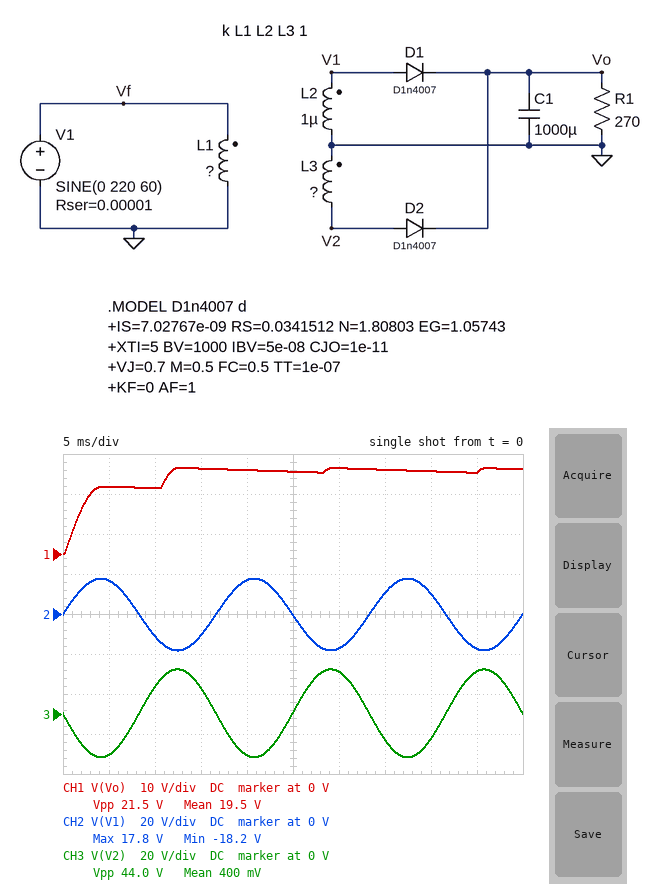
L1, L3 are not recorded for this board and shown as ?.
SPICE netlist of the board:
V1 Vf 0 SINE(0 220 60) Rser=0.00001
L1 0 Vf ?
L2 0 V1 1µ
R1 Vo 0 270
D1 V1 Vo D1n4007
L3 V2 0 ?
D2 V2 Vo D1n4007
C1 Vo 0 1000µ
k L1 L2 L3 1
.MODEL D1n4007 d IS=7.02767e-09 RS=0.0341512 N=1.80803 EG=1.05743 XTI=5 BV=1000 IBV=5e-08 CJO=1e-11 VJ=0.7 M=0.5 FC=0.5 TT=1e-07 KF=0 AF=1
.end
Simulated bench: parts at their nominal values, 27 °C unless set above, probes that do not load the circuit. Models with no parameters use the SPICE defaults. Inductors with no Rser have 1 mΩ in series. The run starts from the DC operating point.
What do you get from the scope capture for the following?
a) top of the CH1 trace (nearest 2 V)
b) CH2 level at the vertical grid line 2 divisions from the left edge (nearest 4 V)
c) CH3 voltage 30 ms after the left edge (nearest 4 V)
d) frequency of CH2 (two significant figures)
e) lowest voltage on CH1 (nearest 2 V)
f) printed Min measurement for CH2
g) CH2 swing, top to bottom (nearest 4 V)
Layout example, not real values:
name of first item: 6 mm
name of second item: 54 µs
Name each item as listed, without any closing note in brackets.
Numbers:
top of the CH1 trace: 22 V
CH2 level at the vertical grid line 2 divisions from the left edge: -12 V
CH3 voltage 30 ms after the left edge: 20 V
frequency of CH2: 60 Hz
lowest voltage on CH1: 0 V
printed Min measurement for CH2: -18.2 V
CH2 swing, top to bottom: 36 V
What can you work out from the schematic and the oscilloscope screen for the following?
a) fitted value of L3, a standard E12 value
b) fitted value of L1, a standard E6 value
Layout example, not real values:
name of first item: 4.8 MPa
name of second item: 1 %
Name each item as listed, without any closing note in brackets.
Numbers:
fitted value of L3, a standard E12 value: 1.5 µH
fitted value of L1, a standard E6 value: 150 µH
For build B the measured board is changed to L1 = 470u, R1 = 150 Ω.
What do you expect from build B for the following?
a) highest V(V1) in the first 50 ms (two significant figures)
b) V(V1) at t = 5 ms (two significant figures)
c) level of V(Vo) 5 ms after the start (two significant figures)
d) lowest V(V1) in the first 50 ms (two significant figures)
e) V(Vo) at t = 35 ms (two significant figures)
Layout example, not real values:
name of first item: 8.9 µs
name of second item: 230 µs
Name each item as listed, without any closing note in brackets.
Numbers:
highest V(V1) in the first 50 ms: 10 V
V(V1) at t = 5 ms: 9.6 V
level of V(Vo) 5 ms after the start: 9.3 V
lowest V(V1) in the first 50 ms: -10 V
V(Vo) at t = 35 ms: 11 V
